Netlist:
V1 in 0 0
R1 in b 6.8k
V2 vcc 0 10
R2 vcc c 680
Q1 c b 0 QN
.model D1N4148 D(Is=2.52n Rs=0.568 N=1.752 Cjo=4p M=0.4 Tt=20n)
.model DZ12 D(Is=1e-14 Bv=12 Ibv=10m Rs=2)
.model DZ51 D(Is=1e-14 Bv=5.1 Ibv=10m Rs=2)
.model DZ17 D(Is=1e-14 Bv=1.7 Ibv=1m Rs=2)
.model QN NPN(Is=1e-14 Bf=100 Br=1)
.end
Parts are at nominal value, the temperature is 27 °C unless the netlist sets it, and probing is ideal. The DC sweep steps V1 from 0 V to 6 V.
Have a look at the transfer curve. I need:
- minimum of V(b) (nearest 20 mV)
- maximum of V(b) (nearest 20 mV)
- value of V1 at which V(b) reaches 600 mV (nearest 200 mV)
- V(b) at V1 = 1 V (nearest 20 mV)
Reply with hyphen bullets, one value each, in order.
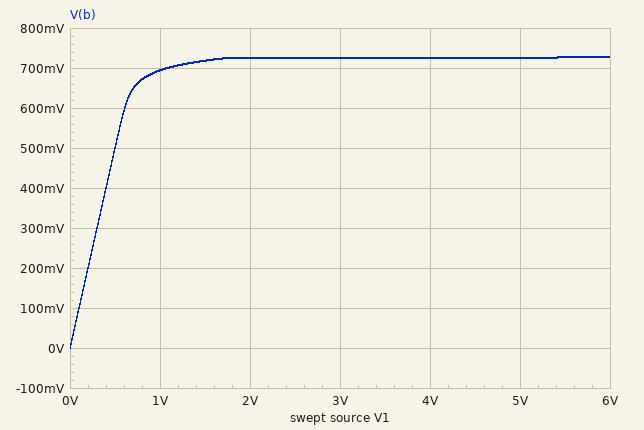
- 0 V
- 720 mV
- 600 mV
- 700 mV
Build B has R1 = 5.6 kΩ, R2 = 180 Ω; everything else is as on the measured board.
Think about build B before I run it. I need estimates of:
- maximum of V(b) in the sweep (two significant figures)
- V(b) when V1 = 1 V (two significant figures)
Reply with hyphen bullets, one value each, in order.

- 760 mV
- 700 mV
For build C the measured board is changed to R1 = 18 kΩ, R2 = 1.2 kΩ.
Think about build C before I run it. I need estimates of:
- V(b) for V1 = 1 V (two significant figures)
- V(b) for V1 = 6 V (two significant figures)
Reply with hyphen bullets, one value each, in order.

- 670 mV
- 710 mV
